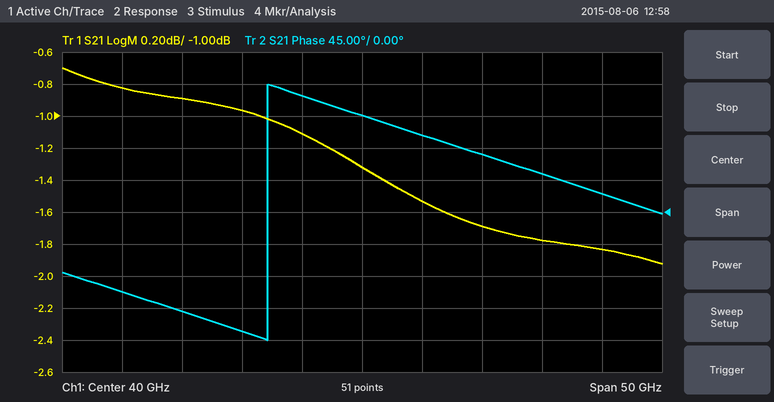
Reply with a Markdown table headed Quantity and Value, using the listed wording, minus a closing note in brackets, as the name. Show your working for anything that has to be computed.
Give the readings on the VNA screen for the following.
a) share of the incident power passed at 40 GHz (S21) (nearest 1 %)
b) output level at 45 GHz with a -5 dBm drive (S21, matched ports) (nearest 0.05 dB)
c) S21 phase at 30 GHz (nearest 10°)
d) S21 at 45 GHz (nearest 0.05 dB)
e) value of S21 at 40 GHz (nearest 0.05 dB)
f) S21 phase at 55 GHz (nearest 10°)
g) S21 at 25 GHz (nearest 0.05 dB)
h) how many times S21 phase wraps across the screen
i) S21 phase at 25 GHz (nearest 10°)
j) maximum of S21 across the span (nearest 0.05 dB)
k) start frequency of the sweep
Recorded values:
| Quantity | Value |
|---|---|
| share of the incident power passed at 40 GHz (S21) | 10^(-1.3/10) ≈ 74 % |
| output level at 45 GHz with a -5 dBm drive (S21, matched ports) | -5 dBm + (-1.55 dB) = -6.55 dBm |
| S21 phase at 30 GHz | -170° |
| S21 at 45 GHz | -1.55 dB |
| value of S21 at 40 GHz | -1.30 dB |
| S21 phase at 55 GHz | 50° |
| S21 at 25 GHz | -0.90 dB |
| how many times S21 phase wraps across the screen | 1 |
| S21 phase at 25 GHz | -140° |
| maximum of S21 across the span | -0.70 dB |
| start frequency of the sweep | 15 GHz |
